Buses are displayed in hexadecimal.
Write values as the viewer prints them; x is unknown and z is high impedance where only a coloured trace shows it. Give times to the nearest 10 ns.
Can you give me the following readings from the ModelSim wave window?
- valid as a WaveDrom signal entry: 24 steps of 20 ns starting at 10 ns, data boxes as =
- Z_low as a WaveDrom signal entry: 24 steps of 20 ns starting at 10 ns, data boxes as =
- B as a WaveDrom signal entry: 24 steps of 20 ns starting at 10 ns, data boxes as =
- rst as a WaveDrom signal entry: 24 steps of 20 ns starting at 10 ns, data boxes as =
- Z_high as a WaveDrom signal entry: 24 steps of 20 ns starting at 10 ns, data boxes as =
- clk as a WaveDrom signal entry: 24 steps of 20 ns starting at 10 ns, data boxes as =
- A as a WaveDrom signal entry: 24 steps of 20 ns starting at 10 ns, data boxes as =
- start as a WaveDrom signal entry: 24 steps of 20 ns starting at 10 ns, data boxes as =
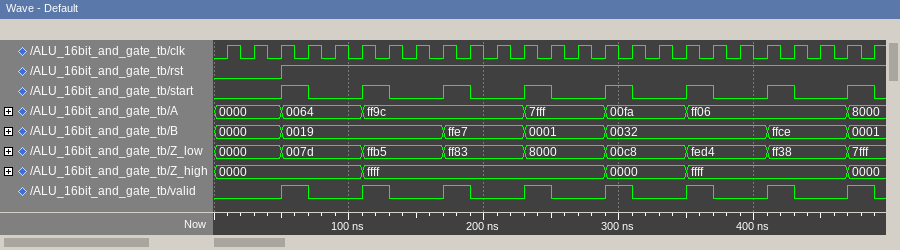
{name: 'valid', wave: '0.10.10.10.10.10.10.10.1'}
{name: 'Z_low', wave: '=.=..=..=..=..=..=..=..=', data: '0000 007d ffb5 ff83 8000 00c8 fed4 ff38 7fff'}
{name: 'B', wave: '=.=.....=..=..=.....=..=', data: '0000 0019 ffe7 0001 0032 ffce 0001'}
{name: 'rst', wave: '0.1.....................'}
{name: 'Z_high', wave: '=....=........=..=.....=', data: '0000 ffff 0000 ffff 0000'}
{name: 'clk', wave: 'p.......................'}
{name: 'A', wave: '=.=..=.....=..=..=.....=', data: '0000 0064 ff9c 7fff 00fa ff06 8000'}
{name: 'start', wave: '0.10.10.10.10.10.10.10.1'}
